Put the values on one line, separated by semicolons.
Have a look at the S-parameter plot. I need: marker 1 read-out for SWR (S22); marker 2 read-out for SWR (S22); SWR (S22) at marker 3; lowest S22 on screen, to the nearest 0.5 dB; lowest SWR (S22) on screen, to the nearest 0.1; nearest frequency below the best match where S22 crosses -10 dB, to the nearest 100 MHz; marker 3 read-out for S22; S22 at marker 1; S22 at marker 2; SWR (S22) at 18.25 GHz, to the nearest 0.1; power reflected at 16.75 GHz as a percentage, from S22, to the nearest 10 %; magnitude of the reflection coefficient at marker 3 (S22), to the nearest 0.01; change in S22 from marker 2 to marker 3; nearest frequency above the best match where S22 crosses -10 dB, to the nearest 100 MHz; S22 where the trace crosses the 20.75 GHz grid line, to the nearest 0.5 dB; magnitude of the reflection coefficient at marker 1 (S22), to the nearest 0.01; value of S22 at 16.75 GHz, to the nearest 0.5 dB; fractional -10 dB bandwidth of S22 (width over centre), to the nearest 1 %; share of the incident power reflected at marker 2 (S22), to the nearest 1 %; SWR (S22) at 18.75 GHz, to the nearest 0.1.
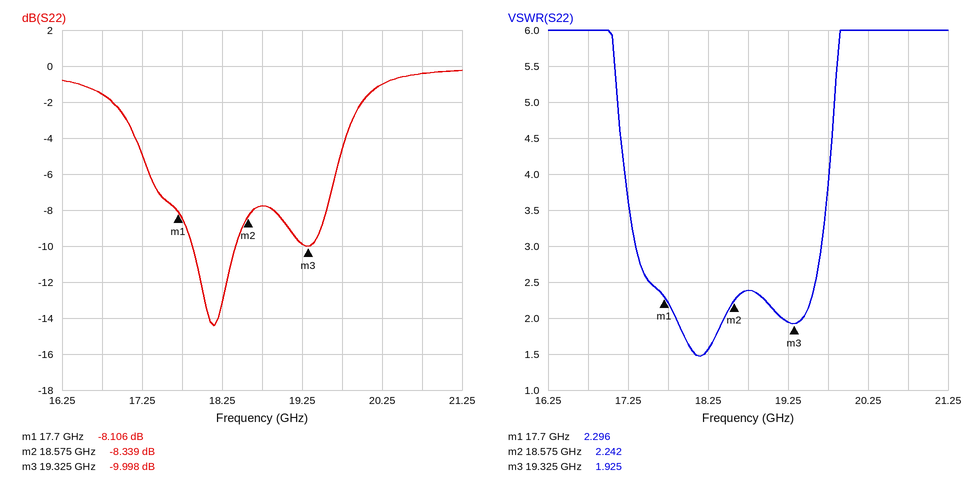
2.296; 2.242; 1.925; -14.5 dB; 1.5; 17.9 GHz; -9.998 dB; -8.106 dB; -8.339 dB; 1.6; 70 %; 0.32; -1.659 dB; 18.4 GHz; -0.5 dB; 0.39; -1.5 dB; 3 %; 15 %; 2.4
